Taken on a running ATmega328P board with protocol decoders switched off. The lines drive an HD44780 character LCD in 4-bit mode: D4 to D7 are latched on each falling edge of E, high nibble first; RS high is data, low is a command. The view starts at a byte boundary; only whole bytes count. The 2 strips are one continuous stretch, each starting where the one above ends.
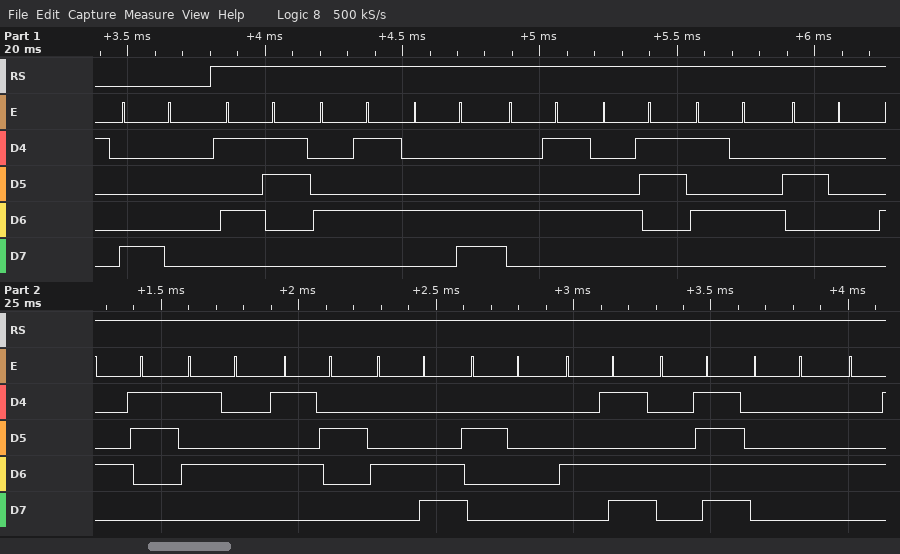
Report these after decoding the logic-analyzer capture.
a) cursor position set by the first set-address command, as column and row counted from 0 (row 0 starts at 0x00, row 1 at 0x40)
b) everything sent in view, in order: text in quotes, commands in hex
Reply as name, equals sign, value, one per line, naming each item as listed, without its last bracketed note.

cursor position set by the first set-address command, as column and row counted from 0 = column 0, row 0
everything sent in view, in order: text in quotes, commands in hex = 0x80 "SELECT CTRL MOD"
